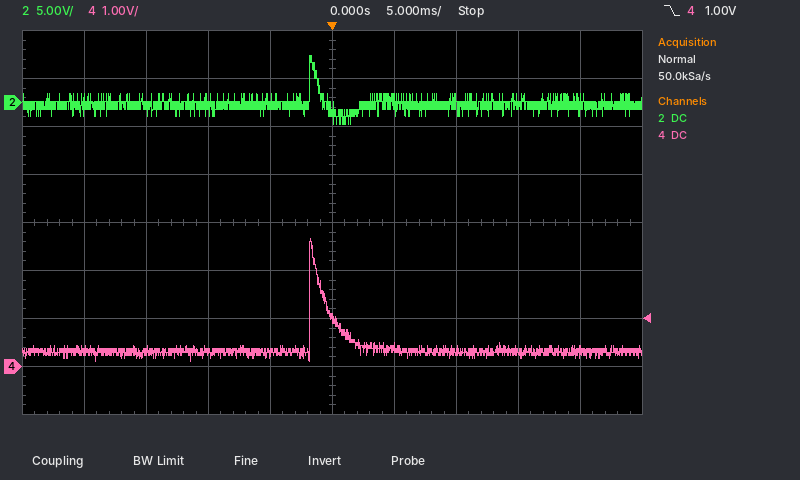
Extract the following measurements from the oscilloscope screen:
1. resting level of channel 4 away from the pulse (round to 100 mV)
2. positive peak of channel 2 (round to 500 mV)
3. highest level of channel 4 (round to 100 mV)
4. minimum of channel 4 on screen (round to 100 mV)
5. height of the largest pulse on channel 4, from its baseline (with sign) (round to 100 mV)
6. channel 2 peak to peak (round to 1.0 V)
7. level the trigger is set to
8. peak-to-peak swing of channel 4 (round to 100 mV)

300 mV
5.0 V
2.7 V
100 mV
+2.4 V
7.0 V
1.00 V
2.6 V
